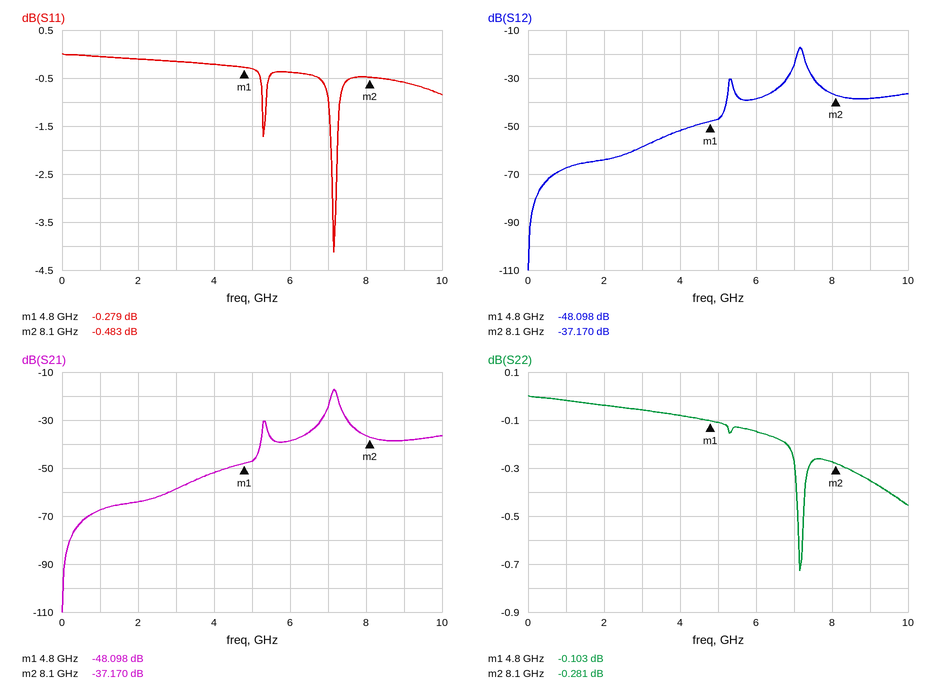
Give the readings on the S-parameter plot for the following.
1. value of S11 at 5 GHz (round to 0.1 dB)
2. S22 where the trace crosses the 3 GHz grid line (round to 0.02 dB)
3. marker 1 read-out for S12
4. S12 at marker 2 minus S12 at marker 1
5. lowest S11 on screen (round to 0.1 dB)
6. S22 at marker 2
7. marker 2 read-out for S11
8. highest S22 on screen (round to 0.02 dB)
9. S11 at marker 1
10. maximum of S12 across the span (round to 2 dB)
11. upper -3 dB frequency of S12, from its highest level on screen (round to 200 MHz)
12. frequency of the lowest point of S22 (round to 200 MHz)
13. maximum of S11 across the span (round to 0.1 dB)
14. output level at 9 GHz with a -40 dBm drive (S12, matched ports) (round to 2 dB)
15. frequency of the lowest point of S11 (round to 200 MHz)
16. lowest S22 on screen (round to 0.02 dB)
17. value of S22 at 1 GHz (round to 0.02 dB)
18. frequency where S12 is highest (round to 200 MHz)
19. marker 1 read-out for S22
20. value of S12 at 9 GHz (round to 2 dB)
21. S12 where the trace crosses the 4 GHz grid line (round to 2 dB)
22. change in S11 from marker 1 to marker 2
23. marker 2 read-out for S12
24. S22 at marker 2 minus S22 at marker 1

-0.3 dB
-0.06 dB
-48.098 dB
10.928 dB
-4.1 dB
-0.281 dB
-0.483 dB
0.00 dB
-0.279 dB
-18 dB
7.2 GHz
7.2 GHz
0.0 dB
-78 dBm
7.2 GHz
-0.72 dB
-0.02 dB
7.2 GHz
-0.103 dB
-38 dB
-52 dB
-0.204 dB
-37.170 dB
-0.178 dB
